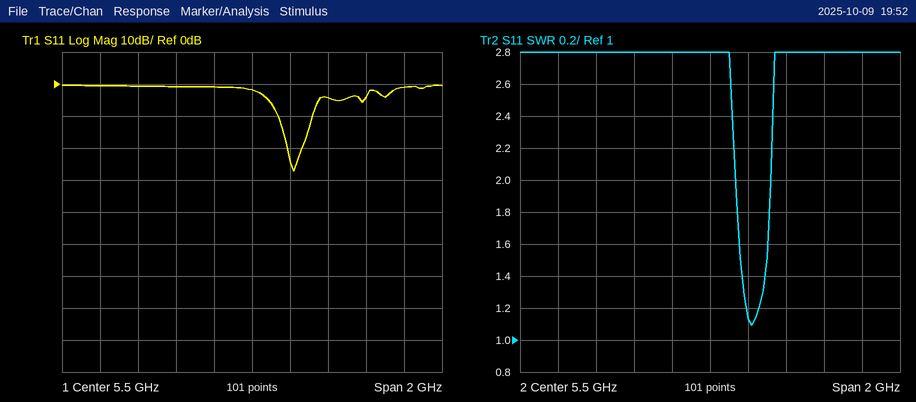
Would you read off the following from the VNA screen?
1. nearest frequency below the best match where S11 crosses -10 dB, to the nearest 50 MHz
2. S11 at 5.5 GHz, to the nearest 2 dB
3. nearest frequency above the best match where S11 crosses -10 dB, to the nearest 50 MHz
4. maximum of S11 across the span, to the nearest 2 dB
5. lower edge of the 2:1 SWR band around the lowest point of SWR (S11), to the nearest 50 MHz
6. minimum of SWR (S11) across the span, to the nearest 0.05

5.65 GHz
-2 dB
5.80 GHz
0 dB
5.65 GHz
1.10
